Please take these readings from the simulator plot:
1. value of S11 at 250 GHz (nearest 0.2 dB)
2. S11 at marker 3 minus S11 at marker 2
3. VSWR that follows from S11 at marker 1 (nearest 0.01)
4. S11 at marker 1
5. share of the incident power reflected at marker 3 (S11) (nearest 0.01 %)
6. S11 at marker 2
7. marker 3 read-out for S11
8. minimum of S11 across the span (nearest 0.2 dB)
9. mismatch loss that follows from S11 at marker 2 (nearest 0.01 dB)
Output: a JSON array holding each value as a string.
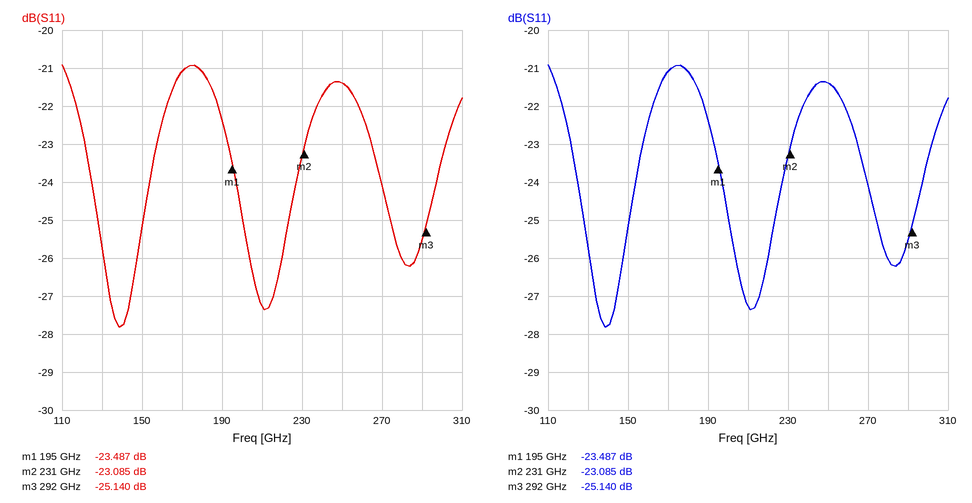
["-21.4 dB", "-2.055 dB", "1.14", "-23.487 dB", "0.31 %", "-23.085 dB", "-25.140 dB", "-27.8 dB", "0.02 dB"]
